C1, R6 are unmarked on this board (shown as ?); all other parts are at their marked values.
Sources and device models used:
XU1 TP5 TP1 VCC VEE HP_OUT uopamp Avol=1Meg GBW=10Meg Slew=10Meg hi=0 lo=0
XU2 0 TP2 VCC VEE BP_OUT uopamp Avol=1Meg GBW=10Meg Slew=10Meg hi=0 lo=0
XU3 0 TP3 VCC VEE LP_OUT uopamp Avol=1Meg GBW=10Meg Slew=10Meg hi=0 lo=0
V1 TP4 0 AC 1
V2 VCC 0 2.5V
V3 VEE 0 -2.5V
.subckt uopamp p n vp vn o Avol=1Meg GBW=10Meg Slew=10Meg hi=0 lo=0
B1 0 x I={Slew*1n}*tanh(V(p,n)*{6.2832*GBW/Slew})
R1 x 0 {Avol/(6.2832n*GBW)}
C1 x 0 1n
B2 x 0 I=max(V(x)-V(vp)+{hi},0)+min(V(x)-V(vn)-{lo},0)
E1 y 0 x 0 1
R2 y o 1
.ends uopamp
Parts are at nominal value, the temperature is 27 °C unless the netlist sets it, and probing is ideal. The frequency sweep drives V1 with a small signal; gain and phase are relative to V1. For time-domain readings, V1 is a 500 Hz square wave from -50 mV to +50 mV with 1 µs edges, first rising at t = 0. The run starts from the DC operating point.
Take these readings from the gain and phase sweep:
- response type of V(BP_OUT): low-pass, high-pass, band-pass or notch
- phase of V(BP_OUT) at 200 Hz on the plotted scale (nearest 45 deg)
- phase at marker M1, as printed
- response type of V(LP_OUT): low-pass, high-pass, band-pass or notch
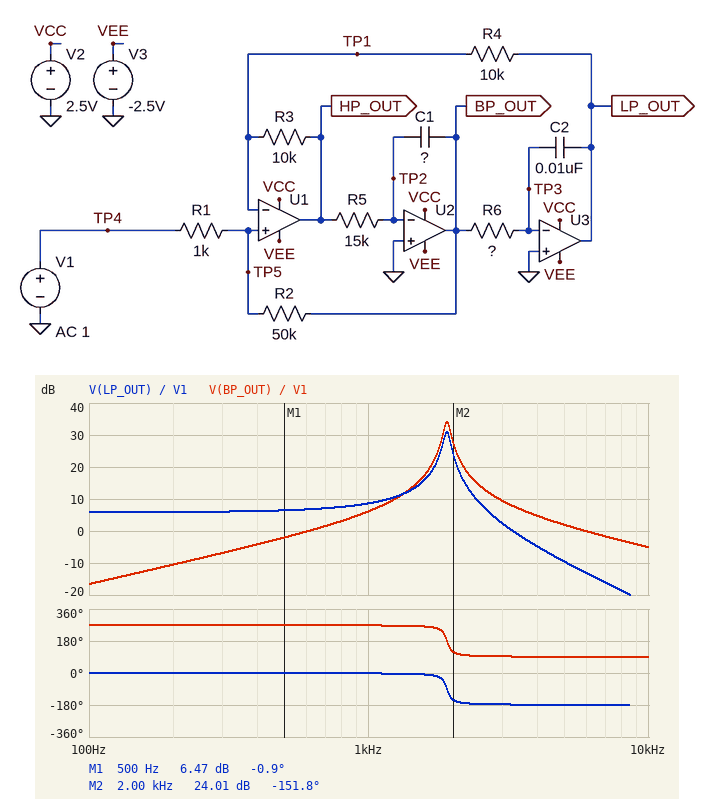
band-pass
270 deg
-0.9 deg
low-pass
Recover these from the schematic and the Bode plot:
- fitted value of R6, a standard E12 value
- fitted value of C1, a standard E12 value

12 kΩ
3.9 nF
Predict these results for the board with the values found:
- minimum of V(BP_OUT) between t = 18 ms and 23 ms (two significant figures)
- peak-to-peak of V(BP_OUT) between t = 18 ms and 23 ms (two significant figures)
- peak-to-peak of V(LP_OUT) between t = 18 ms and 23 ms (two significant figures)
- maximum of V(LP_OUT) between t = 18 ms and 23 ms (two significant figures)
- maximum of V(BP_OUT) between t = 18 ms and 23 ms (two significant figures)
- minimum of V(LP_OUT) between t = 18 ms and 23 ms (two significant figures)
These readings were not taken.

-170 mV
330 mV
420 mV
210 mV
170 mV
-210 mV
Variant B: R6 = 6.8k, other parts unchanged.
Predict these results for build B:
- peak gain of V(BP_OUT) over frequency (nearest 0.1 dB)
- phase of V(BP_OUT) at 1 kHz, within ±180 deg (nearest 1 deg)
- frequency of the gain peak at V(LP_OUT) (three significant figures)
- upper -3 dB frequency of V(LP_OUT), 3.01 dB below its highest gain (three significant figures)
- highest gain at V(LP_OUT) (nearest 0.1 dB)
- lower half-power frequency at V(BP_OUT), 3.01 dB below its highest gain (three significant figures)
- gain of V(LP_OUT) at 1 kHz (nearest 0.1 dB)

34.2 dB
-91 deg
2.52 kHz
2.57 kHz
33.5 dB
2.47 kHz
7.3 dB
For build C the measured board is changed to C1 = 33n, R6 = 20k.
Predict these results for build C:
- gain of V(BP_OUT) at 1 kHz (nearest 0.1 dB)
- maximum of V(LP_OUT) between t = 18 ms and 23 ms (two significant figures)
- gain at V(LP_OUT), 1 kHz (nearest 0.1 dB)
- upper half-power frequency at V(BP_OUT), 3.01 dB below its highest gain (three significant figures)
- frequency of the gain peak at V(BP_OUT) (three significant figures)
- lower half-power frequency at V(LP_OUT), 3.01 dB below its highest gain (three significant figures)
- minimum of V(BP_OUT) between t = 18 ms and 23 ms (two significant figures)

-1.4 dB
2.5 V
-3.4 dB
512 Hz
506 Hz
499 Hz
-1.7 V
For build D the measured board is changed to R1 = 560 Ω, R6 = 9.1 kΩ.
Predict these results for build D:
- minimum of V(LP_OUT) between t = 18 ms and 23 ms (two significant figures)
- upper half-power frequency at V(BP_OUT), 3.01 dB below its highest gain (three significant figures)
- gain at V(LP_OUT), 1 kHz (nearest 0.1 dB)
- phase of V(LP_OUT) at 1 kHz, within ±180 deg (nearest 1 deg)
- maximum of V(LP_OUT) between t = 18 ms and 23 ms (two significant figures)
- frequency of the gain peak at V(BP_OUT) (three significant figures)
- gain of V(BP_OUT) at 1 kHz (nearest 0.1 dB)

-220 mV
2.21 kHz
8.0 dB
-1 deg
220 mV
2.18 kHz
3.1 dB
